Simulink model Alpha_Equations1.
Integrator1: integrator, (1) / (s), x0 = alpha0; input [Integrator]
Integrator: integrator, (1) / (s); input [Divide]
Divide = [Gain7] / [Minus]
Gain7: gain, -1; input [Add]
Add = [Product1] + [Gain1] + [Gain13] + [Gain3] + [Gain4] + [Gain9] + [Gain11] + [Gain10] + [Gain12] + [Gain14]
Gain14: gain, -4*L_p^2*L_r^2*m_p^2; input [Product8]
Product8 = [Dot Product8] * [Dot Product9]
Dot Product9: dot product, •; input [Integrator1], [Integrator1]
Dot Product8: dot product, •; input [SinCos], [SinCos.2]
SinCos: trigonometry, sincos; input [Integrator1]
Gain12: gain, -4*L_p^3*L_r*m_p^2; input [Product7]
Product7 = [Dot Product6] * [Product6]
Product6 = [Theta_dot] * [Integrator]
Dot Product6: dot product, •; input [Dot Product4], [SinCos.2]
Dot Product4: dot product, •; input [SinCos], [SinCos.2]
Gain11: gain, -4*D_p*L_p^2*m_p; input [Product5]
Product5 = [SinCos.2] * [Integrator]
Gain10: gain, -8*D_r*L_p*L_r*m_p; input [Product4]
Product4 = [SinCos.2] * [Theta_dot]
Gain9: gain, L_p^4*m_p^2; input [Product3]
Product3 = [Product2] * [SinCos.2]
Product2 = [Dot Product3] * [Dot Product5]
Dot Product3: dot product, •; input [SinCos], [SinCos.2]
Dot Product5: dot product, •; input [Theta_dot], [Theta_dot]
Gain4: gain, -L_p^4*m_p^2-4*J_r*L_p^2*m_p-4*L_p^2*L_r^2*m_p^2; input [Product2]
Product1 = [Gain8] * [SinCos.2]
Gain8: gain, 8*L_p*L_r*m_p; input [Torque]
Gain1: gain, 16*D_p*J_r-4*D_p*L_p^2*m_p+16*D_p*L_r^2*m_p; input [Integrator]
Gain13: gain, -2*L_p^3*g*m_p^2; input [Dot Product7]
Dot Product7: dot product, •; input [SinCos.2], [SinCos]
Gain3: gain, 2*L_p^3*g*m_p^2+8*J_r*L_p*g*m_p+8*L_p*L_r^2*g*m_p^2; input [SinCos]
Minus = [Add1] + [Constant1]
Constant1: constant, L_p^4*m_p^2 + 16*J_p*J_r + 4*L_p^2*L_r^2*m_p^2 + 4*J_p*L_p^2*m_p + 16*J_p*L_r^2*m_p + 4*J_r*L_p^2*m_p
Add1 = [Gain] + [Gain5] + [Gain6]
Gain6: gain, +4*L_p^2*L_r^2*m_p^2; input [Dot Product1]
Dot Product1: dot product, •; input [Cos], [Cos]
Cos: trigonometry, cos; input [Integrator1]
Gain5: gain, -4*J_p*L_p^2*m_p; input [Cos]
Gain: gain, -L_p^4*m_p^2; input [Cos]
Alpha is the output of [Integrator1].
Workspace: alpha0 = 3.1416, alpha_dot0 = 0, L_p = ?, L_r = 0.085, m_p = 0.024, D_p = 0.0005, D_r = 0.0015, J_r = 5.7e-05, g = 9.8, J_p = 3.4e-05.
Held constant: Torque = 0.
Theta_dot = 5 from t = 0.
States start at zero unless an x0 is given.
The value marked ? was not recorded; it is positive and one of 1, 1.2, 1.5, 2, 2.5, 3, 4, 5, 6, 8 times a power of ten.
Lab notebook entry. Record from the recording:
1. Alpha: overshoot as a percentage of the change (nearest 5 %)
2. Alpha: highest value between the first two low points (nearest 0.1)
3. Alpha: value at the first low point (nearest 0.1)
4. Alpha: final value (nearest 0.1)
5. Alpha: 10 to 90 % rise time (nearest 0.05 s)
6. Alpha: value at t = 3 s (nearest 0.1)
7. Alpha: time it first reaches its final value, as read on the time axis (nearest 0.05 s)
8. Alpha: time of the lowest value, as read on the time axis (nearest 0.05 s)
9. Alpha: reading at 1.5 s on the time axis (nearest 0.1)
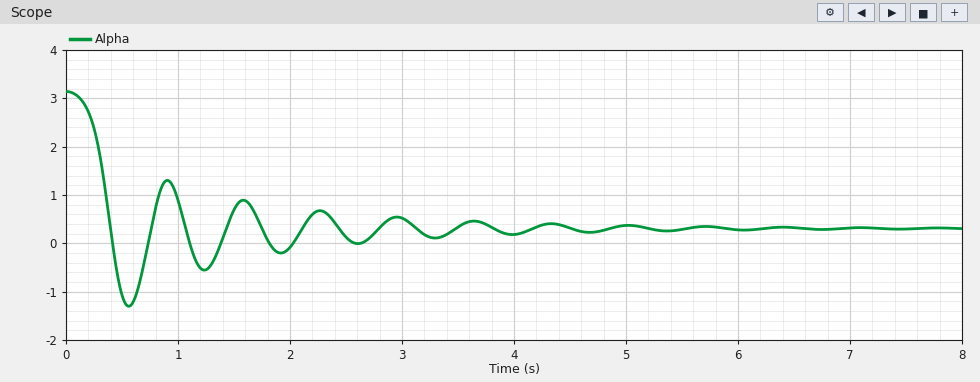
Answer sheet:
55 %
1.3
-1.3
0.3
0.20 s
0.5
0.40 s
0.55 s
0.7
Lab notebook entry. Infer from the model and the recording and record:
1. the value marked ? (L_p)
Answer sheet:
0.1
